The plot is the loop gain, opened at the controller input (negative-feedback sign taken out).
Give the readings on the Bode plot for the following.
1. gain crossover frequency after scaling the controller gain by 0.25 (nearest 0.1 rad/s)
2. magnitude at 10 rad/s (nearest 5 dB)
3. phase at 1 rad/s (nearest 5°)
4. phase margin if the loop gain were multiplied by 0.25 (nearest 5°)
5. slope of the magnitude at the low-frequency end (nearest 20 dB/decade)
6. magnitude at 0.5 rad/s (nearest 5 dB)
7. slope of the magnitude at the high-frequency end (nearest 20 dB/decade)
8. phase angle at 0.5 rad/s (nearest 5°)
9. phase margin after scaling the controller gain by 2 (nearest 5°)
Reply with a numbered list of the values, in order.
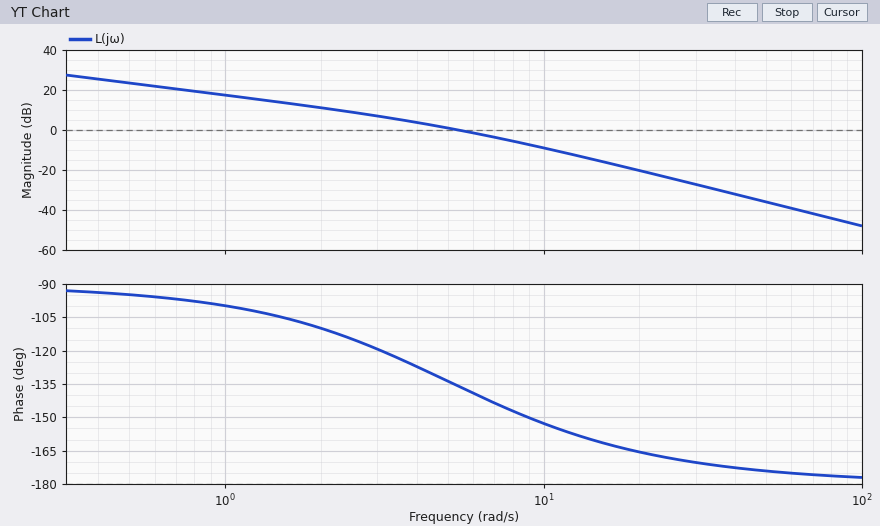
1. 1.8 rad/s
2. -10 dB
3. -100°
4. 70°
5. -20 dB/decade
6. 25 dB
7. -40 dB/decade
8. -95°
9. 30°
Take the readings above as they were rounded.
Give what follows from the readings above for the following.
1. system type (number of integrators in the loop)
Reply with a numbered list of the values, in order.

1. 1
